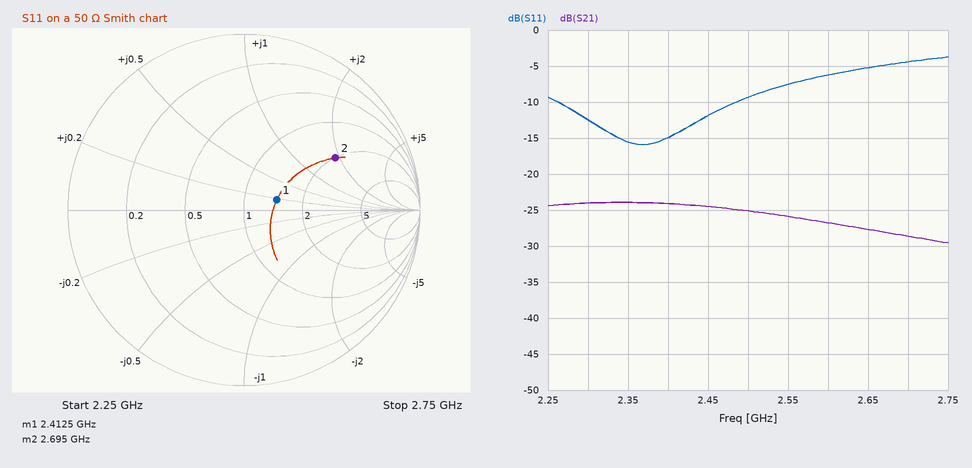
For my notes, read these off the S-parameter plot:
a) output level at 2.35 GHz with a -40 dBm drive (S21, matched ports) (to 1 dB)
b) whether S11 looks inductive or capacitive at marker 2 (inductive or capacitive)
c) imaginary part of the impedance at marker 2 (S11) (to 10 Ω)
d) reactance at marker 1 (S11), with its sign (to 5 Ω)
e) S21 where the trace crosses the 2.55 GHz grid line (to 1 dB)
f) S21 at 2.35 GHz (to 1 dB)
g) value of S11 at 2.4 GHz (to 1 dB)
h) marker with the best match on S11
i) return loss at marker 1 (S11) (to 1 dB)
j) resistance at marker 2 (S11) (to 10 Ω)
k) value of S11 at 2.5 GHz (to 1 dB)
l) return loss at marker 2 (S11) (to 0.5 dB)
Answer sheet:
-64 dBm
inductive
+90 Ω
+10 Ω
-26 dB
-24 dB
-15 dB
marker 1
14 dB
100 Ω
-9 dB
4.5 dB
